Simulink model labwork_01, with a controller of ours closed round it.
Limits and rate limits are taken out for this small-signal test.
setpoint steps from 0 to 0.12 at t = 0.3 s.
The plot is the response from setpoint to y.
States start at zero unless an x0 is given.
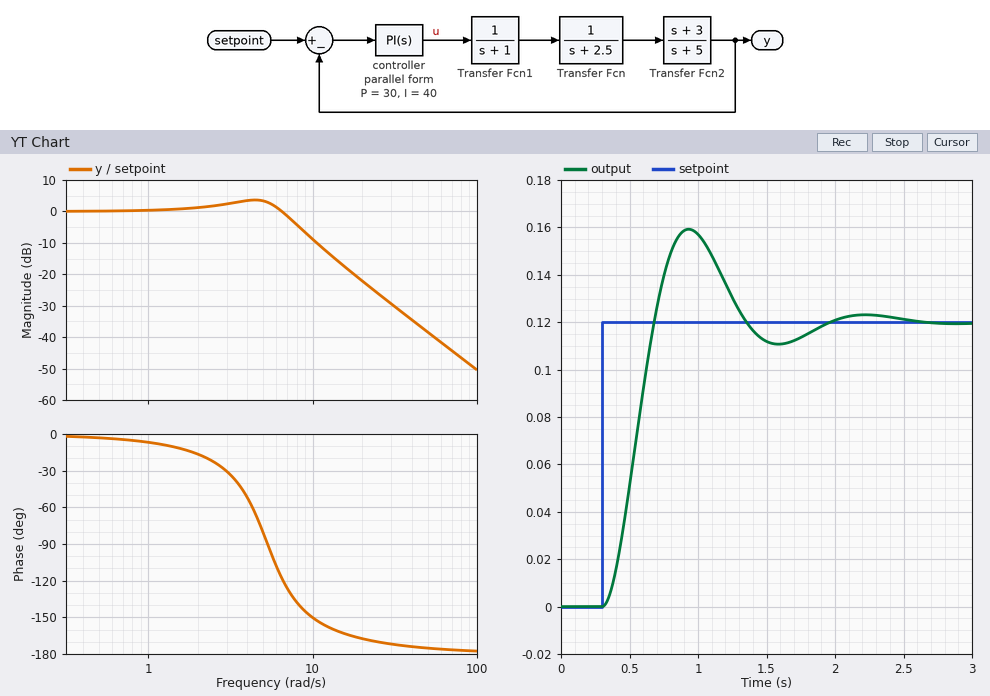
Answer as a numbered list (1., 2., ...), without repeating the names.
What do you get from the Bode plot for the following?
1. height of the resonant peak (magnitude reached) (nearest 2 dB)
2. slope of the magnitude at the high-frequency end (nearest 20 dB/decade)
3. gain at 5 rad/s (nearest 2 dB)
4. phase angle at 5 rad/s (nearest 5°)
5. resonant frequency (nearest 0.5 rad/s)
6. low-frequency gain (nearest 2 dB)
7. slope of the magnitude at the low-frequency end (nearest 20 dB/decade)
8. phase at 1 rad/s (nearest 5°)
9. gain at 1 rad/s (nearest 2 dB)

1. 4 dB
2. -40 dB/decade
3. 4 dB
4. -80°
5. 4.5 rad/s
6. 0 dB
7. 0 dB/decade
8. -5°
9. 0 dB
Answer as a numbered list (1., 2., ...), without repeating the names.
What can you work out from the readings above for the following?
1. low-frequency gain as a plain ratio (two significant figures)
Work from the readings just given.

1. 1.0
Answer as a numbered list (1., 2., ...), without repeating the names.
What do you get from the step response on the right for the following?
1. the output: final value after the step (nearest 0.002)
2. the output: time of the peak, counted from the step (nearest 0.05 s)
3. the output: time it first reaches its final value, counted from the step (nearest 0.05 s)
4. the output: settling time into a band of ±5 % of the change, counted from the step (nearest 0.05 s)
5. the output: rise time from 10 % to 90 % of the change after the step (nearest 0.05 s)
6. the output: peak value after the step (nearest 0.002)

1. 0.120
2. 0.65 s
3. 0.40 s
4. 1.45 s
5. 0.25 s
6. 0.160
